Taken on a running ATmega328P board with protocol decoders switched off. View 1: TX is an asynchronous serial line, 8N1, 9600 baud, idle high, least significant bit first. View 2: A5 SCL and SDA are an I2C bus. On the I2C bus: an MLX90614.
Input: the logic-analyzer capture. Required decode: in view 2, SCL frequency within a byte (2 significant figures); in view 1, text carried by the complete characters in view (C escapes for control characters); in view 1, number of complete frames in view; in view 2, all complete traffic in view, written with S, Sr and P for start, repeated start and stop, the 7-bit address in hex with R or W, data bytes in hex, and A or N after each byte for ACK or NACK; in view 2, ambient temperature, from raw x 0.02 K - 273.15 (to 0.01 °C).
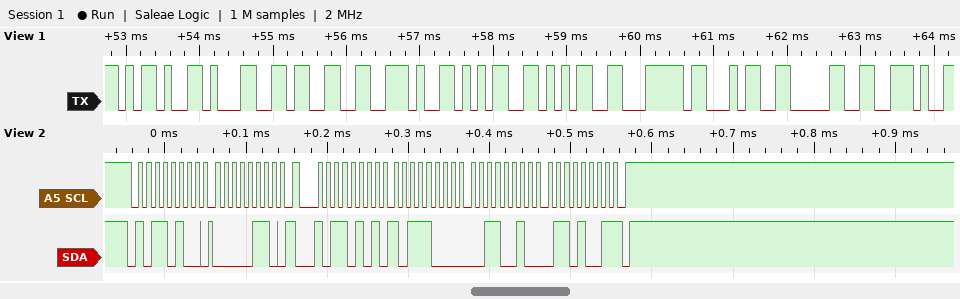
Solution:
100 kHz
"-13.55|40."
10
S 5AW A 06 A Sr 5AR A B8 A 32 A 69 N P
-13.47 °C
